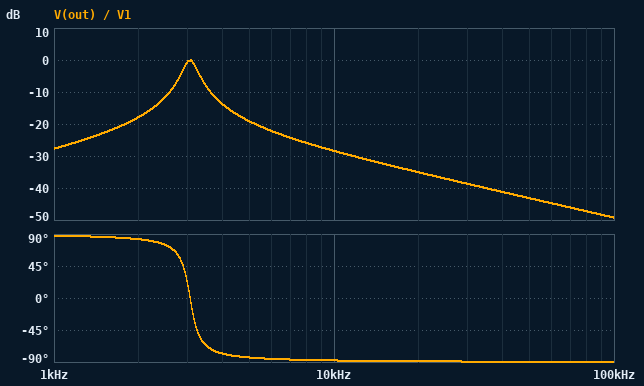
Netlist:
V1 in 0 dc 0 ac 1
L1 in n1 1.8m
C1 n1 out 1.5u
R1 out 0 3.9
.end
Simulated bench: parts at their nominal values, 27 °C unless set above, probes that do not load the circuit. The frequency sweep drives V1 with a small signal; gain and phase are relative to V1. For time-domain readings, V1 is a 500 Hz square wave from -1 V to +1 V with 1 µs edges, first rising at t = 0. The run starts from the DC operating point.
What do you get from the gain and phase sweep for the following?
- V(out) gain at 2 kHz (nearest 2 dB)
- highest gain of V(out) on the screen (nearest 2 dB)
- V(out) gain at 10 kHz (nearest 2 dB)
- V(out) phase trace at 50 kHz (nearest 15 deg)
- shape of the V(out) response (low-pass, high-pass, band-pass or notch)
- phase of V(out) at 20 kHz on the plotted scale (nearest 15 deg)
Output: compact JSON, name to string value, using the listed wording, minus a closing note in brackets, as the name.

{"V(out) gain at 2 kHz": "-18 dB", "highest gain of V(out) on the screen": "0 dB", "V(out) gain at 10 kHz": "-28 dB", "V(out) phase trace at 50 kHz": "-90 deg", "shape of the V(out) response": "band-pass", "phase of V(out) at 20 kHz on the plotted scale": "-90 deg"}
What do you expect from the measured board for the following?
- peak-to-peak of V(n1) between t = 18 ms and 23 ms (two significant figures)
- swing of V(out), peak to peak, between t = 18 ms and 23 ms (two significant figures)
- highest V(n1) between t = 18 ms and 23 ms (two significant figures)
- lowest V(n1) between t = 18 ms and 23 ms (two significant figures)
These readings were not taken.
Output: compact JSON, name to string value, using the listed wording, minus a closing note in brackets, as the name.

{"peak-to-peak of V(n1) between t = 18 ms and 23 ms": "4.5 V", "swing of V(out), peak to peak, between t = 18 ms and 23 ms": "310 mV", "highest V(n1) between t = 18 ms and 23 ms": "2.3 V", "lowest V(n1) between t = 18 ms and 23 ms": "-2.3 V"}
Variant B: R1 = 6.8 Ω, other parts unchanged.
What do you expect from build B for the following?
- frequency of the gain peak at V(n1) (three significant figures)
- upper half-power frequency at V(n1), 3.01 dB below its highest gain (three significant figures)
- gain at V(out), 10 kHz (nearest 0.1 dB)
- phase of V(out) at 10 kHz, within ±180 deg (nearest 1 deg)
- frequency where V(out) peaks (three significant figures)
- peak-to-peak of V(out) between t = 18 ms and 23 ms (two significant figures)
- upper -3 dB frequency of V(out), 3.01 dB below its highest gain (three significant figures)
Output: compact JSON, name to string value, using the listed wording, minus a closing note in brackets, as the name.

{"frequency of the gain peak at V(n1)": "3.03 kHz", "upper half-power frequency at V(n1), 3.01 dB below its highest gain": "3.32 kHz", "gain at V(out), 10 kHz": "-23.6 dB", "phase of V(out) at 10 kHz, within ±180 deg": "-86 deg", "frequency where V(out) peaks": "3.06 kHz", "peak-to-peak of V(out) between t = 18 ms and 23 ms": "590 mV", "upper -3 dB frequency of V(out), 3.01 dB below its highest gain": "3.38 kHz"}
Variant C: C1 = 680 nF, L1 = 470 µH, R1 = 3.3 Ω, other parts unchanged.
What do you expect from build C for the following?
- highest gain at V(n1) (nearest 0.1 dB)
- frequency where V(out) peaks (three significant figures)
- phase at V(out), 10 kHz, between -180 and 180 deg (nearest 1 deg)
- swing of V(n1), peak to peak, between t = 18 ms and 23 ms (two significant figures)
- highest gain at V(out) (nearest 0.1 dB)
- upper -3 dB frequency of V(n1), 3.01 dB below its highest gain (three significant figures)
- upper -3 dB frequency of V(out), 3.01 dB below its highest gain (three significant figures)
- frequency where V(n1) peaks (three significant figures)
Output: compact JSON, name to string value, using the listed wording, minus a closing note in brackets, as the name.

{"highest gain at V(n1)": "18.1 dB", "frequency where V(out) peaks": "8.90 kHz", "phase at V(out), 10 kHz, between -180 and 180 deg": "-62 deg", "swing of V(n1), peak to peak, between t = 18 ms and 23 ms": "5.3 V", "highest gain at V(out)": "0 dB", "upper -3 dB frequency of V(n1), 3.01 dB below its highest gain": "9.41 kHz", "upper -3 dB frequency of V(out), 3.01 dB below its highest gain": "9.48 kHz", "frequency where V(n1) peaks": "8.87 kHz"}
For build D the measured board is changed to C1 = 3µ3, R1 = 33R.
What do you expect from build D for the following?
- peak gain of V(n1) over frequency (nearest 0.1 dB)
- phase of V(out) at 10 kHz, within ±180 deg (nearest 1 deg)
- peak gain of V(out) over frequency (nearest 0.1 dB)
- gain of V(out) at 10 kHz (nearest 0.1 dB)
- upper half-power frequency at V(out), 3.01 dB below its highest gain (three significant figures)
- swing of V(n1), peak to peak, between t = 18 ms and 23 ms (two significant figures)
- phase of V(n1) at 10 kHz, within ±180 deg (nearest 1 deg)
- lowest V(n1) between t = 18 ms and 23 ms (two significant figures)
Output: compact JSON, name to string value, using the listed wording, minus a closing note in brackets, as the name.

{"peak gain of V(n1) over frequency": "2.1 dB", "phase of V(out) at 10 kHz, within ±180 deg": "-73 deg", "peak gain of V(out) over frequency": "0 dB", "gain of V(out) at 10 kHz": "-10.7 dB", "upper half-power frequency at V(out), 3.01 dB below its highest gain": "3.99 kHz", "swing of V(n1), peak to peak, between t = 18 ms and 23 ms": "2.8 V", "phase of V(n1) at 10 kHz, within ±180 deg": "-81 deg", "lowest V(n1) between t = 18 ms and 23 ms": "-1.4 V"}
